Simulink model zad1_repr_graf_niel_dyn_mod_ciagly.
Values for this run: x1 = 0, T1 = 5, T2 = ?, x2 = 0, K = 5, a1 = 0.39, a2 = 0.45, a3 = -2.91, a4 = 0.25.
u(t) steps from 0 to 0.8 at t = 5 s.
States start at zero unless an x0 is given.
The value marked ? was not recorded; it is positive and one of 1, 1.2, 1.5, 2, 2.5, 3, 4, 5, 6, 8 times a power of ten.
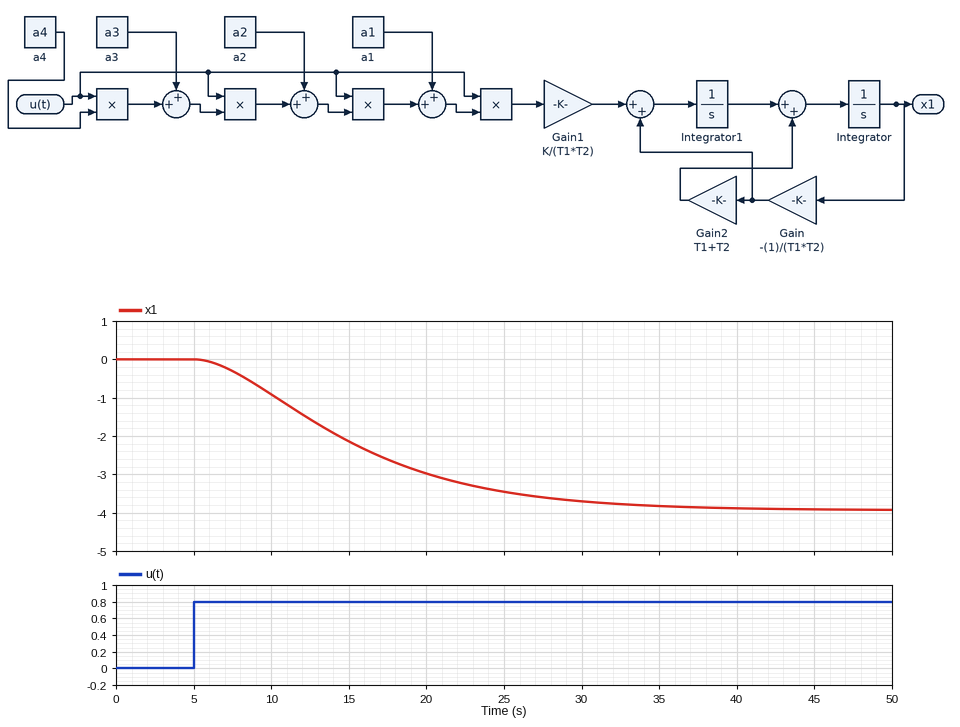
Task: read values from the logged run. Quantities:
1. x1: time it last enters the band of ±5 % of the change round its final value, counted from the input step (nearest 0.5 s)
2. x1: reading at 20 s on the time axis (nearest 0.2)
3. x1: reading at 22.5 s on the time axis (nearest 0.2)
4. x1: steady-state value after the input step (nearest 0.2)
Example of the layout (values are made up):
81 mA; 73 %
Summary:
26.0 s; -3.0; -3.2; -4.0
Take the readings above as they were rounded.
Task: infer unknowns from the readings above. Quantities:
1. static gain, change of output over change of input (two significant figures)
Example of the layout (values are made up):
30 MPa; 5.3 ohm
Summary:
-5.0
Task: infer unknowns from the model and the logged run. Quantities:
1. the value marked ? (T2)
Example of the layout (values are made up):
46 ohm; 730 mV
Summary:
6
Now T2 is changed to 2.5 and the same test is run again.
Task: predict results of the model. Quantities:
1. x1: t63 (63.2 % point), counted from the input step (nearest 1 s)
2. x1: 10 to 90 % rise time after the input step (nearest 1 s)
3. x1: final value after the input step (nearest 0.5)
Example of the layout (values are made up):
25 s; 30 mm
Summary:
8 s; 13 s; -4.0
